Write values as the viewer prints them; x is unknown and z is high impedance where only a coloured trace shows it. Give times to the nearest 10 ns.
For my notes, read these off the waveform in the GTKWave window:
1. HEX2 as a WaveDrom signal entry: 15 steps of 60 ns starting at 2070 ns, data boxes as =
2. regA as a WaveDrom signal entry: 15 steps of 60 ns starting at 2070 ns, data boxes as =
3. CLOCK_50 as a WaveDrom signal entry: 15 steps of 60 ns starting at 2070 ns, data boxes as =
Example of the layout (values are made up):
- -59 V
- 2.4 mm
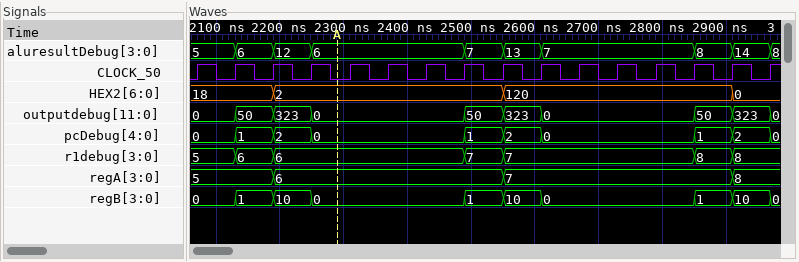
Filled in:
- {name: 'HEX2', wave: '=.=.....=.....=', data: '18 2 120 0'}
- {name: 'regA', wave: '=.=.....=.....=', data: '5 6 7 8'}
- {name: 'CLOCK_50', wave: 'p..............'}
